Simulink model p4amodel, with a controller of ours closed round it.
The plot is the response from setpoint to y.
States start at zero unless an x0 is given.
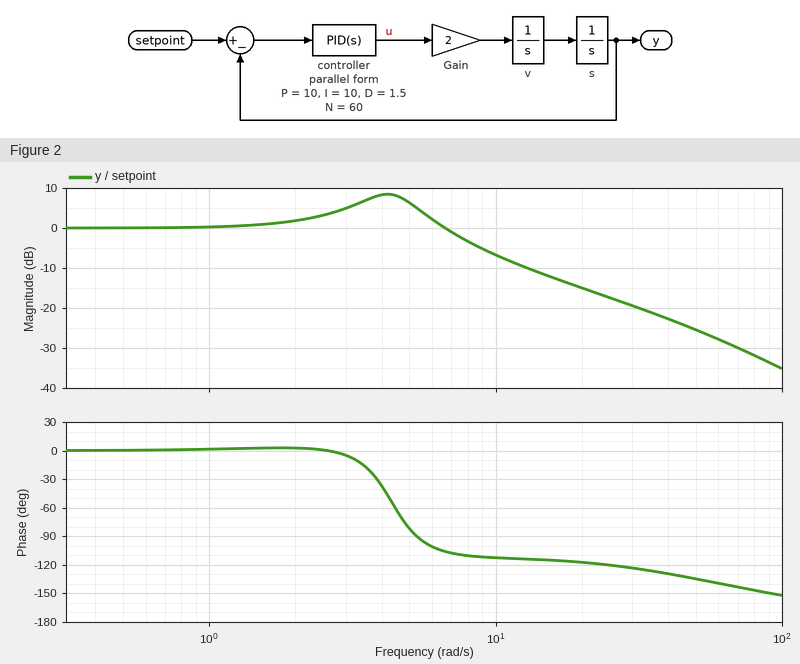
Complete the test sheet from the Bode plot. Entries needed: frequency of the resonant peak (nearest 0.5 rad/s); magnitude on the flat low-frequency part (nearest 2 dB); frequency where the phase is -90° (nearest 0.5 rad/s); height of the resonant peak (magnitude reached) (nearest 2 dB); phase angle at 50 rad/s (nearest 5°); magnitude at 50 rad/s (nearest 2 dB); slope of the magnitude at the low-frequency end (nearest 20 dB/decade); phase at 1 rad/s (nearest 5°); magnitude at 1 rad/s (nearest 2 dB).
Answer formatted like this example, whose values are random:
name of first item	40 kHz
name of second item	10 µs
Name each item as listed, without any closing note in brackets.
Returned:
frequency of the resonant peak	4.0 rad/s
magnitude on the flat low-frequency part	0 dB
frequency where the phase is -90°	5.5 rad/s
height of the resonant peak (magnitude reached)	8 dB
phase angle at 50 rad/s	-135°
magnitude at 50 rad/s	-26 dB
slope of the magnitude at the low-frequency end	0 dB/decade
phase at 1 rad/s	0°
magnitude at 1 rad/s	0 dB
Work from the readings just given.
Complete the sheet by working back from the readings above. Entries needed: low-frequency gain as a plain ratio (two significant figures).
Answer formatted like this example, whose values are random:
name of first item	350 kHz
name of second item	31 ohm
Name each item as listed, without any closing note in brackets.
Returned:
low-frequency gain as a plain ratio	1.0
